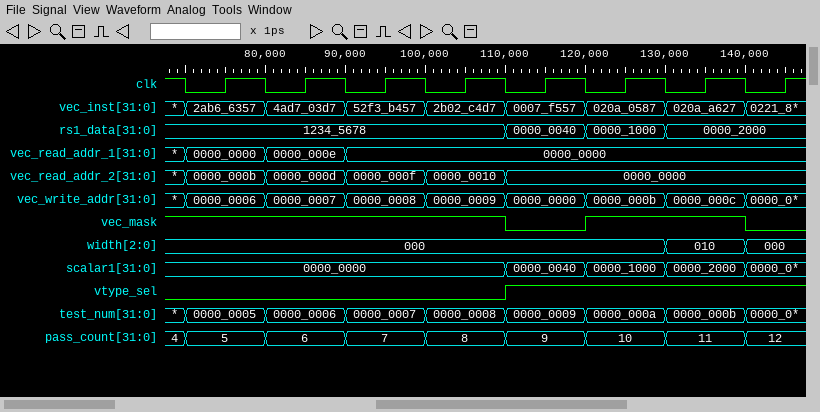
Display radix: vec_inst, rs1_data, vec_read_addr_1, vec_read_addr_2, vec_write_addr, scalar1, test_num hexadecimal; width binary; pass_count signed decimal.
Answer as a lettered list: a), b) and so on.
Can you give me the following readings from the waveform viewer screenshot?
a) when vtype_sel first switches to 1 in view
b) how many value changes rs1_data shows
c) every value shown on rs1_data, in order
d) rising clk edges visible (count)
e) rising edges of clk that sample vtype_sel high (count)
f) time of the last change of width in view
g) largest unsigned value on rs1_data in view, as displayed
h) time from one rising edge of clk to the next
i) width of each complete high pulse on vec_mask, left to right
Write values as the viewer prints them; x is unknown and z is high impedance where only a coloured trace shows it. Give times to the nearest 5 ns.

a) 110 ns
b) 3
c) 1234_5678, 0000_0040, 0000_1000, 0000_2000
d) 8
e) 4
f) 140 ns
g) 1234_5678
h) 10 ns
i) 20 ns
